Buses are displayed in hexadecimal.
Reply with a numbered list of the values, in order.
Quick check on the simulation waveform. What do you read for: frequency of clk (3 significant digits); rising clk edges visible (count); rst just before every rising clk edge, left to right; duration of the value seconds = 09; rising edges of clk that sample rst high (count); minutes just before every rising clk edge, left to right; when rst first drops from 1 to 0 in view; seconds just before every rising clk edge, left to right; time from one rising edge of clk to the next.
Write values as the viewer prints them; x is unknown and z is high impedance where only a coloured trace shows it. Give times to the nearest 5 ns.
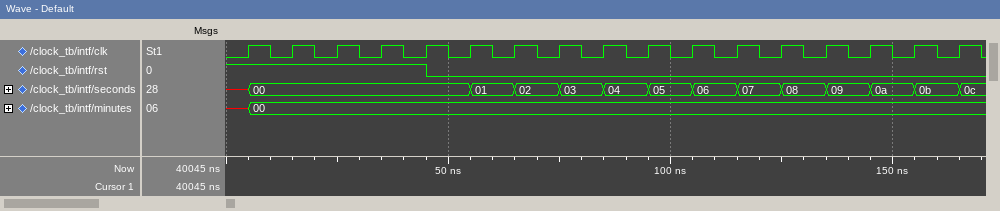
1. 100 MHz
2. 17
3. 1 1 1 1 1 0 0 0 0 0 0 0 0 0 0 0 0
4. 10 ns
5. 5
6. x, 00, 00, 00, 00, 00, 00, 00, 00, 00, 00, 00, 00, 00, 00, 00, 00
7. 45 ns
8. x, 00, 00, 00, 00, 00, 01, 02, 03, 04, 05, 06, 07, 08, 09, 0a, 0b
9. 10 ns
